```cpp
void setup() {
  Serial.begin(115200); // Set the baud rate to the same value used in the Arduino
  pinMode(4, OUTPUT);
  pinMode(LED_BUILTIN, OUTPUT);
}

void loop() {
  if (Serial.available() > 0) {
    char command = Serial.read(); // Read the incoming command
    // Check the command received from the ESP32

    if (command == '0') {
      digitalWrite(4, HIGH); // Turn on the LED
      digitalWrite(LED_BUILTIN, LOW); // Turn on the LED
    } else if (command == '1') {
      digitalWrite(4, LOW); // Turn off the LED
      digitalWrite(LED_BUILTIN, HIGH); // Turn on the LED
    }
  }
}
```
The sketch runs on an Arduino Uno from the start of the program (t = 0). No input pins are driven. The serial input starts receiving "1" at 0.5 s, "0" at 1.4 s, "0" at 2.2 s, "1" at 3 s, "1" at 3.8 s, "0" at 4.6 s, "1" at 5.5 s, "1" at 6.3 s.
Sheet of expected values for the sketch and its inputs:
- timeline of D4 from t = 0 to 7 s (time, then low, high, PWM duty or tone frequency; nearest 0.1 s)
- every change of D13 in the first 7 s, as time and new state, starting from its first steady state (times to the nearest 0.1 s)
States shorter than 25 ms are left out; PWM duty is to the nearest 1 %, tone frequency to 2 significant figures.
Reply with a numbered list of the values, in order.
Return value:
1. 0 s low; 1.4 s high; 3 s low; 4.6 s high; 5.5 s low
2. 0 s low; 0.5 s high; 1.4 s low; 3 s high; 4.6 s low; 5.5 s high
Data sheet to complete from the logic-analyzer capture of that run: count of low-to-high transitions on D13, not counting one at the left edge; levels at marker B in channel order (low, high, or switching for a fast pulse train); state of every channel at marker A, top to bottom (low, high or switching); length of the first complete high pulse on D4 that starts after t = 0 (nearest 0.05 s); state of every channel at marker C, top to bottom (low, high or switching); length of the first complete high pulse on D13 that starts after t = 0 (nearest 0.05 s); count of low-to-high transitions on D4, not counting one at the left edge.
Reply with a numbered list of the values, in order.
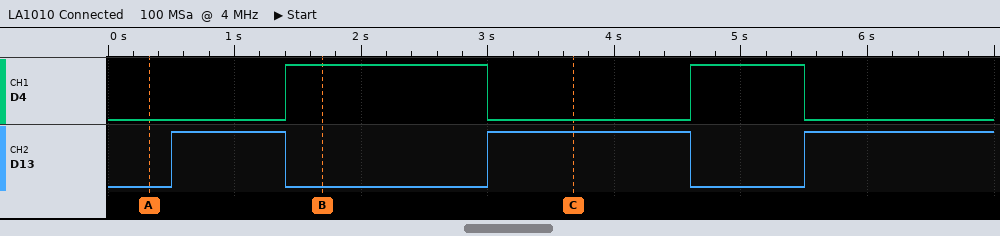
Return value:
1. 3
2. D4 high, D13 low
3. D4 low, D13 low
4. 1.60 s
5. D4 low, D13 high
6. 0.90 s
7. 2
